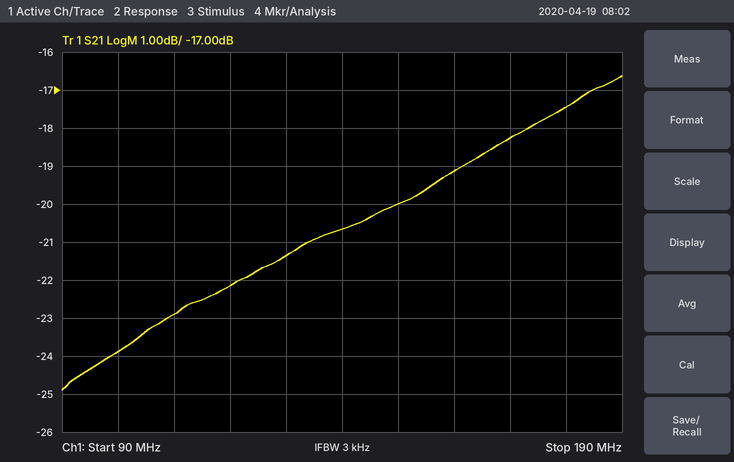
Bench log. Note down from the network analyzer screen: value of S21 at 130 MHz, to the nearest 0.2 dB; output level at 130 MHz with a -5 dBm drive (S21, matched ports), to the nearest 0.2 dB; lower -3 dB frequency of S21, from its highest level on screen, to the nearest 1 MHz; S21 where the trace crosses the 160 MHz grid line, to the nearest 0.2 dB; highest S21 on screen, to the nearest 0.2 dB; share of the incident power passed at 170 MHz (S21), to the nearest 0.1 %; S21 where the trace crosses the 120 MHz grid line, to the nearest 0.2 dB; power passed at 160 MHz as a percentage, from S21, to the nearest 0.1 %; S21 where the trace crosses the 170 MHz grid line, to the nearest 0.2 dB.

-21.4 dB
-26.4 dBm
155 MHz
-19.2 dB
-16.6 dB
1.5 %
-22.2 dB
1.2 %
-18.2 dB
